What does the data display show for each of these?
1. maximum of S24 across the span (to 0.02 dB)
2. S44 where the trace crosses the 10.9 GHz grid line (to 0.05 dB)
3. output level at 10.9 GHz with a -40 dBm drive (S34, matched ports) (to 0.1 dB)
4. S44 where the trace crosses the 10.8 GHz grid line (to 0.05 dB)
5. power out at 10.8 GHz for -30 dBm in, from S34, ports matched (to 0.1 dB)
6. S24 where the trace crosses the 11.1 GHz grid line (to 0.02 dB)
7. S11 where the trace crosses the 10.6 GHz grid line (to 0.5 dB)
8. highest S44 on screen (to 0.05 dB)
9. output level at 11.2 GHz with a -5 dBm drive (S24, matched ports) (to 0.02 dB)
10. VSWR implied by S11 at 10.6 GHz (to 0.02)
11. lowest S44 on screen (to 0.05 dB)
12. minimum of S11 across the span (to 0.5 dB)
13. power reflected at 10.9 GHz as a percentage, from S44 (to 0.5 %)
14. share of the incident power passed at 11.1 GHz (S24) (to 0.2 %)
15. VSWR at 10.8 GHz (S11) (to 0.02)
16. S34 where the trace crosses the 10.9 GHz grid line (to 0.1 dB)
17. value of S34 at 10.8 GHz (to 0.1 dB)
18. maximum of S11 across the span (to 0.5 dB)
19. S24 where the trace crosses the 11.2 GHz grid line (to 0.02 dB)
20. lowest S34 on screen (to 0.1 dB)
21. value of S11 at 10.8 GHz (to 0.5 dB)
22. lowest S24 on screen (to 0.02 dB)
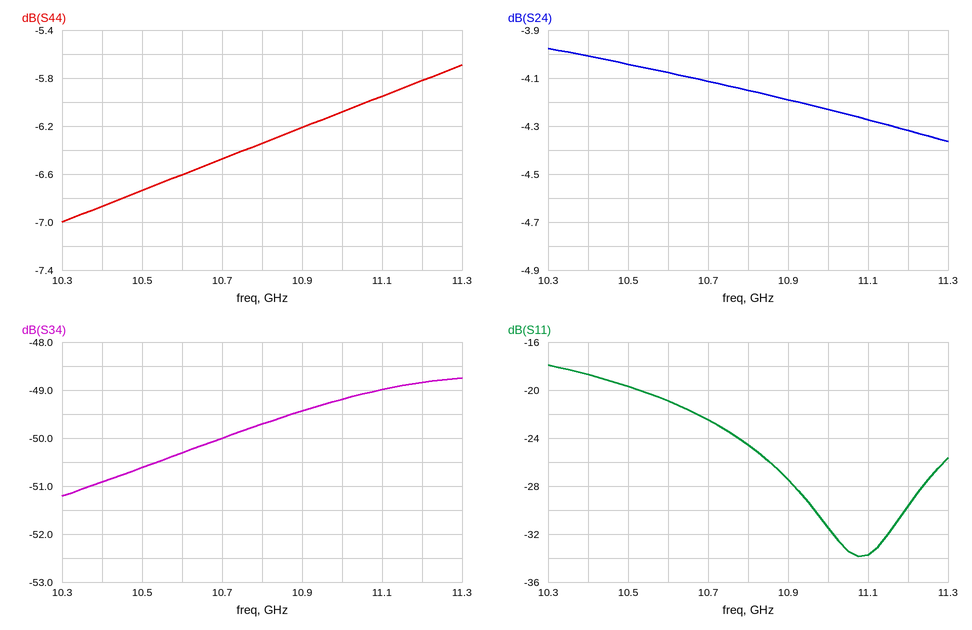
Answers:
-3.98 dB
-6.20 dB
-89.4 dBm
-6.35 dB
-79.7 dBm
-4.28 dB
-21.0 dB
-5.70 dB
-9.32 dBm
1.20
-7.00 dB
-34.0 dB
24.0 %
37.4 %
1.12
-49.4 dB
-49.7 dB
-18.0 dB
-4.32 dB
-51.2 dB
-24.5 dB
-4.36 dB
